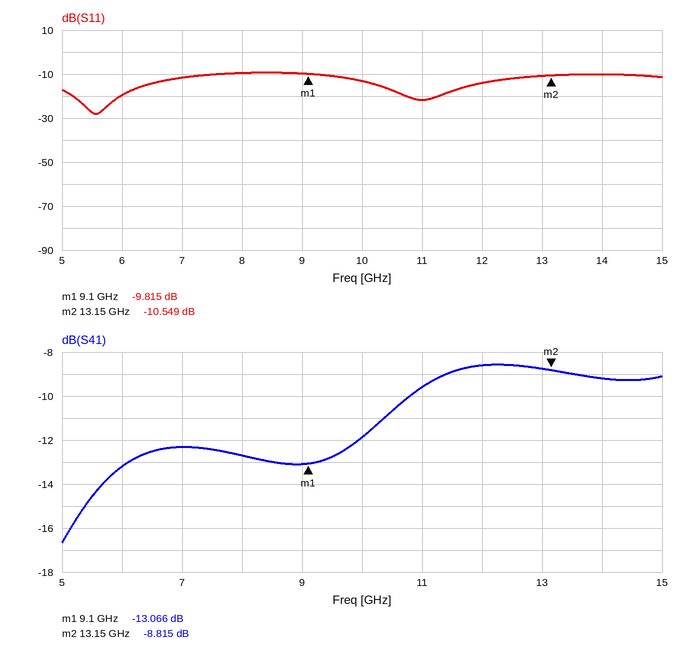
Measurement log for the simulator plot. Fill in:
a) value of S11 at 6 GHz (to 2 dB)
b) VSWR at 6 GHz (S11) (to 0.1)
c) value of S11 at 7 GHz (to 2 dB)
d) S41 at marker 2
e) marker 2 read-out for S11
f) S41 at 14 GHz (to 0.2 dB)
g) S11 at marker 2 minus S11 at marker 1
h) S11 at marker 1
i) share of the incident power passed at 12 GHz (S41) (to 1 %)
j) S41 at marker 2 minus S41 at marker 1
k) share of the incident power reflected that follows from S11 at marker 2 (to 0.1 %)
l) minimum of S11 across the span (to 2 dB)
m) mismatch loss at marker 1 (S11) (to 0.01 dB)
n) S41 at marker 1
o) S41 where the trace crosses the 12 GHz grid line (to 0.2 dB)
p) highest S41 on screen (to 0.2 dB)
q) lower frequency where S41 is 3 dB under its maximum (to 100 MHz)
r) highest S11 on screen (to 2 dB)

-20 dB
1.2
-12 dB
-8.815 dB
-10.549 dB
-9.2 dB
-0.734 dB
-9.815 dB
14 %
4.251 dB
8.8 %
-28 dB
0.48 dB
-13.066 dB
-8.6 dB
-8.6 dB
10.1 GHz
-10 dB
